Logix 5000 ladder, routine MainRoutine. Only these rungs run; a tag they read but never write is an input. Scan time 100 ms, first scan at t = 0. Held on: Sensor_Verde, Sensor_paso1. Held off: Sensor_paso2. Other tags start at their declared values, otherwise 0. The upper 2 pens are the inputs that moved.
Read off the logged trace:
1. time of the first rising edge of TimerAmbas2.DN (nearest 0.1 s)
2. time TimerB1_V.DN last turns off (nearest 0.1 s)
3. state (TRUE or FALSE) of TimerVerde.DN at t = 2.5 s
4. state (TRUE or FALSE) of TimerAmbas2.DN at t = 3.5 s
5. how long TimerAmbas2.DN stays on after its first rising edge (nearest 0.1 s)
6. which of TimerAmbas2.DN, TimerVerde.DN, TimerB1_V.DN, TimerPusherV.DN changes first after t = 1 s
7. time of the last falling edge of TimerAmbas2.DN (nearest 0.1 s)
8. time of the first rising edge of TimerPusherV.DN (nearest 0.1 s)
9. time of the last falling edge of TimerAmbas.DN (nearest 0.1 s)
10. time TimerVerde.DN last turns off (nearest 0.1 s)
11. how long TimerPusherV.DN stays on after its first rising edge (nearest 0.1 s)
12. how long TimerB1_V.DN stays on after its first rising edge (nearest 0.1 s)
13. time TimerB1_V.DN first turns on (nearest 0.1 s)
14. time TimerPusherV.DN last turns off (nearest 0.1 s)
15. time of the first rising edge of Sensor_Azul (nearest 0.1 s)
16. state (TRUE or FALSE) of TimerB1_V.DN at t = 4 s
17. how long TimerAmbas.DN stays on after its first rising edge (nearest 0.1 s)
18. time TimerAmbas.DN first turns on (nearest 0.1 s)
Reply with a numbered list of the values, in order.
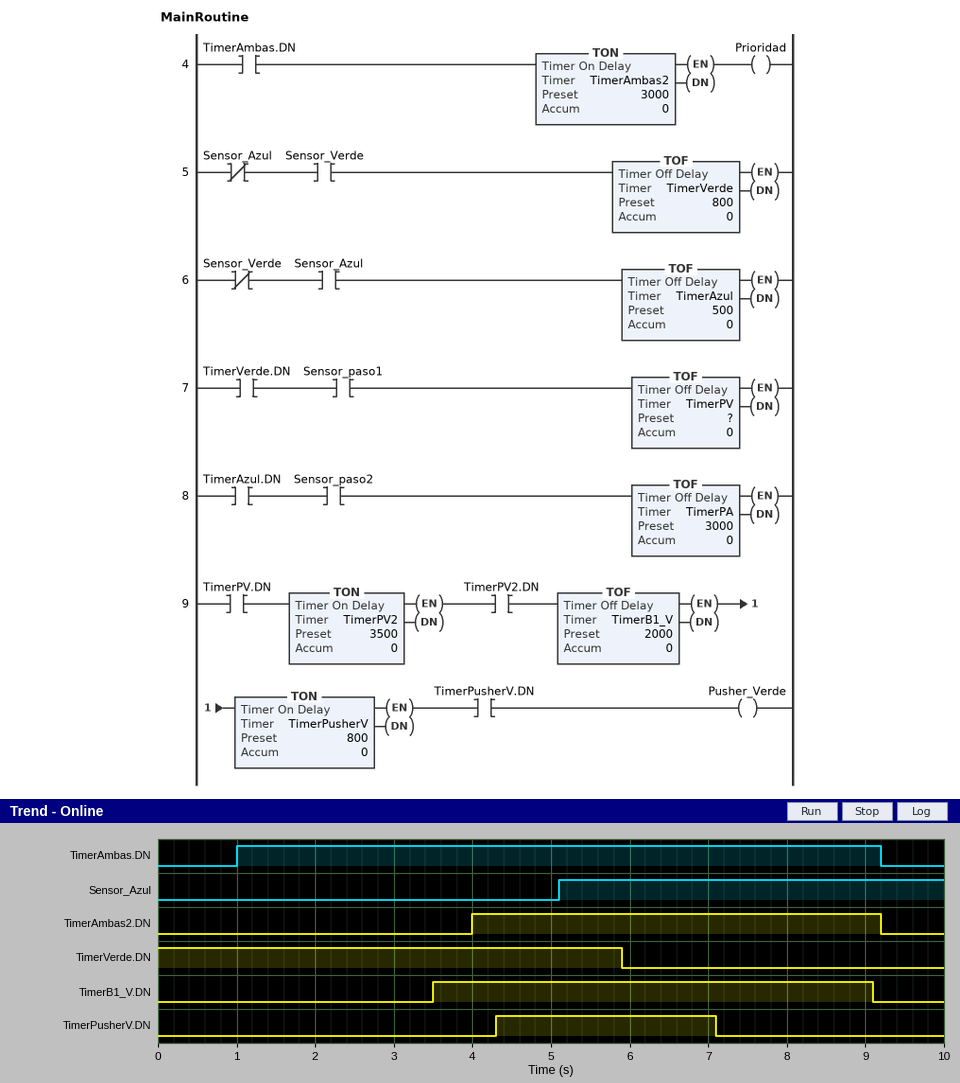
1. 4.0 s
2. 9.1 s
3. TRUE
4. FALSE
5. 5.2 s
6. TimerB1_V.DN
7. 9.2 s
8. 4.3 s
9. 9.2 s
10. 5.9 s
11. 2.8 s
12. 5.6 s
13. 3.5 s
14. 7.1 s
15. 5.1 s
16. TRUE
17. 8.2 s
18. 1.0 s
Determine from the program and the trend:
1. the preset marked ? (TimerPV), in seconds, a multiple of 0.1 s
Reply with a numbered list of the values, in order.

1. 1.2 s
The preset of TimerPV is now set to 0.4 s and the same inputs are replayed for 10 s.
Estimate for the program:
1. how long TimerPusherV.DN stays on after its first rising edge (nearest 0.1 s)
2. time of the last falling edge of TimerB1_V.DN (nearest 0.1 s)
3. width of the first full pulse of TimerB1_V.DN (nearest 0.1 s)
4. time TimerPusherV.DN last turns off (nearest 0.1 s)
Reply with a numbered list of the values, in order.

1. 2.0 s
2. 8.3 s
3. 4.8 s
4. 6.3 s
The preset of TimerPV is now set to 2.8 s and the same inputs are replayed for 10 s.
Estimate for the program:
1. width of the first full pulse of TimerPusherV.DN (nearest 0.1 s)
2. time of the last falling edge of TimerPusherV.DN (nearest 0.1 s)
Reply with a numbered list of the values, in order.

1. 4.4 s
2. 8.7 s
